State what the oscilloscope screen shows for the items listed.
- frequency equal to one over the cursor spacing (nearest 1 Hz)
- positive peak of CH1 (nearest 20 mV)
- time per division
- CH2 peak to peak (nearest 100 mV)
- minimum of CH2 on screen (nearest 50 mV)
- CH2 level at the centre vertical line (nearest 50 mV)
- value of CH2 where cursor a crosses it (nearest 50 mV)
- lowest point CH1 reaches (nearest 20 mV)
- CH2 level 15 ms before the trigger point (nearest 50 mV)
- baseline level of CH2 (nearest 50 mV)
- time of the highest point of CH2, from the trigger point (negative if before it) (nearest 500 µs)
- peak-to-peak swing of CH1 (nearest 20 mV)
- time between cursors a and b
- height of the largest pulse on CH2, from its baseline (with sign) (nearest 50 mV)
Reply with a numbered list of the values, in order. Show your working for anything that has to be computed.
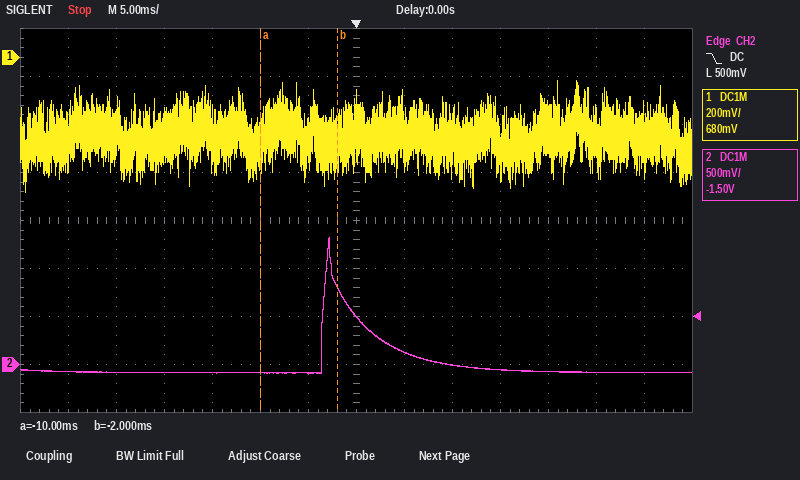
1. 1 / 8.0 ms ≈ 125 Hz
2. -100 mV
3. 5 ms
4. 1.40 V
5. -100 mV
6. 500 mV
7. -100 mV
8. -560 mV
9. -100 mV
10. -100 mV
11. -3.0 ms
12. -100 mV − (-560 mV) = 460 mV
13. -2 ms − (-10 ms) = 8.0 ms
14. +1.40 V
